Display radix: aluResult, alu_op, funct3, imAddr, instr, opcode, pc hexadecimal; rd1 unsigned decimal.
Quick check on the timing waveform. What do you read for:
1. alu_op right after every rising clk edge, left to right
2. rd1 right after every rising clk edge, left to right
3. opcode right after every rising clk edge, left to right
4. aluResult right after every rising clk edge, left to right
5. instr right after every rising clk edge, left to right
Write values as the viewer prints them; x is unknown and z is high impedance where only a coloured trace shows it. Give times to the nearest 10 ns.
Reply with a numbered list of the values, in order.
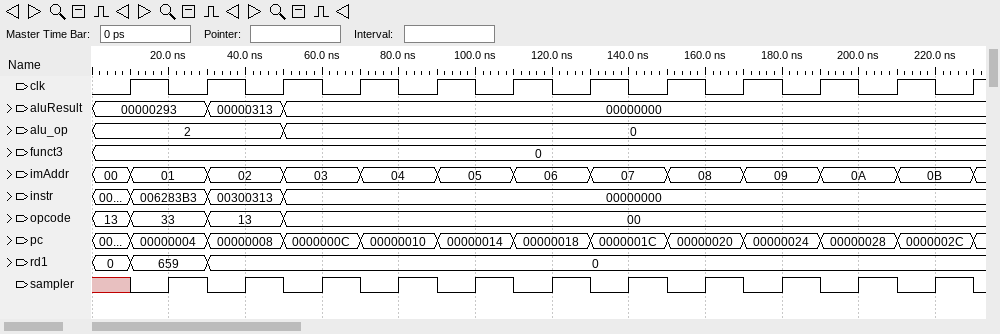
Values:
1. 2, 2, 0, 0, 0, 0, 0, 0, 0, 0, 0, 0
2. 659, 0, 0, 0, 0, 0, 0, 0, 0, 0, 0, 0
3. 33, 13, 00, 00, 00, 00, 00, 00, 00, 00, 00, 00
4. 00000293, 00000313, 00000000, 00000000, 00000000, 00000000, 00000000, 00000000, 00000000, 00000000, 00000000, 00000000
5. 006283B3, 00300313, 00000000, 00000000, 00000000, 00000000, 00000000, 00000000, 00000000, 00000000, 00000000, 00000000
